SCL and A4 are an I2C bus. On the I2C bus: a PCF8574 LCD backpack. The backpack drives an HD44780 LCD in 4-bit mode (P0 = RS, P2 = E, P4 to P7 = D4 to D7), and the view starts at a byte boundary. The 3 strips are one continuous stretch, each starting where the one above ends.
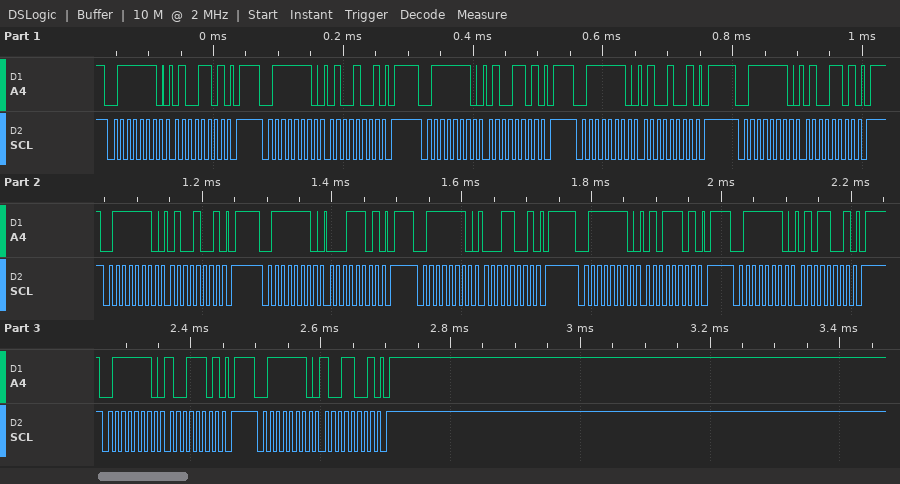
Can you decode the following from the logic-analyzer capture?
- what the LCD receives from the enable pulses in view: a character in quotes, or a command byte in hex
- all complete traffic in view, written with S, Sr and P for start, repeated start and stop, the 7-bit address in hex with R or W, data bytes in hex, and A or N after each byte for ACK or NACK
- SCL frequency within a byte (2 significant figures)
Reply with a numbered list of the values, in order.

1. 'D' 'A' 'Y'
2. S 3FW A 4D A P S 3FW A 49 A P S 3FW A 4D A P S 3FW A 49 A P S 3FW A 4D A P S 3FW A 49 A P S 3FW A 1D A P S 3FW A 19 A P S 3FW A 5D A P S 3FW A 59 A P S 3FW A 9D A P S 3FW A 99 A P
3. 100 kHz
